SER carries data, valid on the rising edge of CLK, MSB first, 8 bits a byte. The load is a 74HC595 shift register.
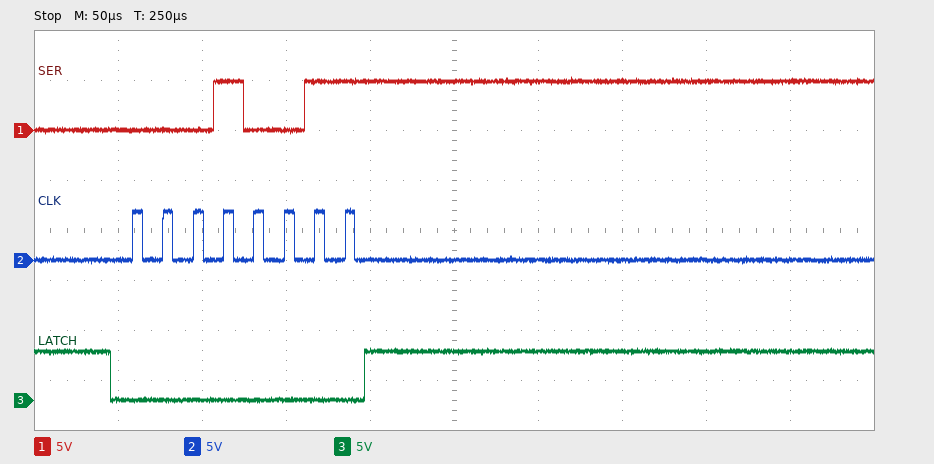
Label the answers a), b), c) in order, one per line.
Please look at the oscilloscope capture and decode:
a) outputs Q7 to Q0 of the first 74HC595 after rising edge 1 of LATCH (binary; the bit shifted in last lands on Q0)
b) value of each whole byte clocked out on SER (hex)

a) 00010011
b) 0x13
